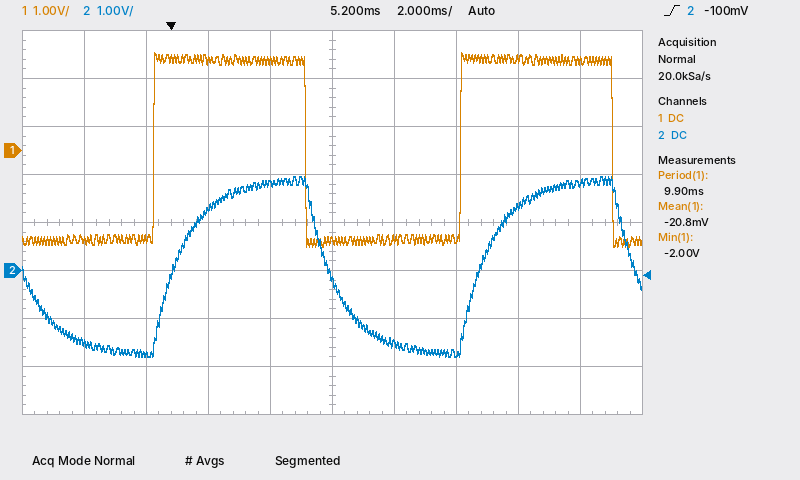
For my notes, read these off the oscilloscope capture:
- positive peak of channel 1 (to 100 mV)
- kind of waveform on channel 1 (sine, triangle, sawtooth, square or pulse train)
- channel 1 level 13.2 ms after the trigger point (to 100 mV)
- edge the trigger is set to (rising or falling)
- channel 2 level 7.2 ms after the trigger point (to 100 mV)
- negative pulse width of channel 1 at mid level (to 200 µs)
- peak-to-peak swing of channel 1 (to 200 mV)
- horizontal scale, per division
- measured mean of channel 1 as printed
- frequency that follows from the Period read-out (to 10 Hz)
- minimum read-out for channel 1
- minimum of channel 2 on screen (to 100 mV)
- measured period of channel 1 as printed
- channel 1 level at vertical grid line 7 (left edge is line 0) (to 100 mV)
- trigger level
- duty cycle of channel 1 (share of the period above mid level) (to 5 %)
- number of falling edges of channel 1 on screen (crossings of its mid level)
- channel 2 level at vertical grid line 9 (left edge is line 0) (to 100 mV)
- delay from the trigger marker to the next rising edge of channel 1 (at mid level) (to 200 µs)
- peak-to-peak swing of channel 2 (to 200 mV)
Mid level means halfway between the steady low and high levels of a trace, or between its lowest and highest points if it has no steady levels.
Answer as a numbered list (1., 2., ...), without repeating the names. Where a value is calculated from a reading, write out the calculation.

1. 2.0 V
2. square
3. 1.9 V
4. rising
5. -1.5 V
6. 5.0 ms
7. 4.0 V
8. 2 ms
9. -20.8 mV
10. 1 / 9.90 ms ≈ 101 Hz, so 100 Hz to the nearest 10 Hz
11. -2.00 V
12. -1.8 V
13. 9.90 ms
14. -1.8 V
15. -100 mV
16. 50 %
17. 2
18. 1.8 V
19. 9.4 ms
20. 3.8 V
